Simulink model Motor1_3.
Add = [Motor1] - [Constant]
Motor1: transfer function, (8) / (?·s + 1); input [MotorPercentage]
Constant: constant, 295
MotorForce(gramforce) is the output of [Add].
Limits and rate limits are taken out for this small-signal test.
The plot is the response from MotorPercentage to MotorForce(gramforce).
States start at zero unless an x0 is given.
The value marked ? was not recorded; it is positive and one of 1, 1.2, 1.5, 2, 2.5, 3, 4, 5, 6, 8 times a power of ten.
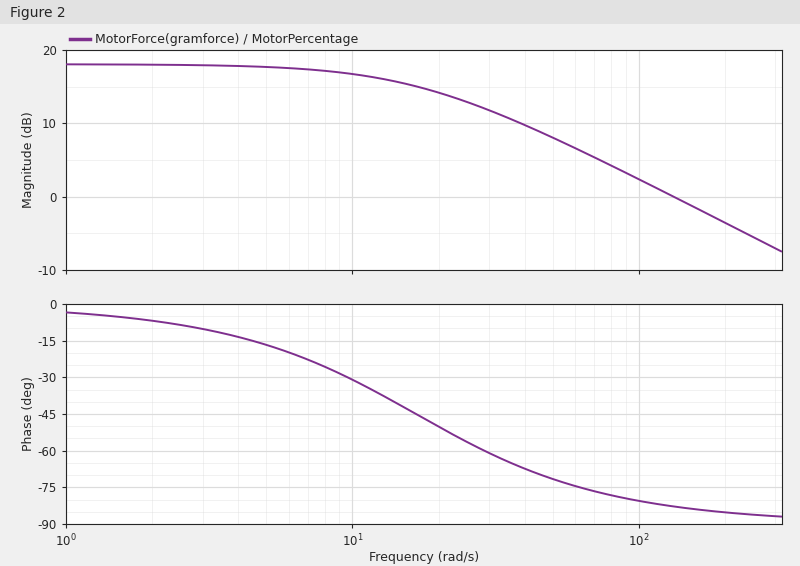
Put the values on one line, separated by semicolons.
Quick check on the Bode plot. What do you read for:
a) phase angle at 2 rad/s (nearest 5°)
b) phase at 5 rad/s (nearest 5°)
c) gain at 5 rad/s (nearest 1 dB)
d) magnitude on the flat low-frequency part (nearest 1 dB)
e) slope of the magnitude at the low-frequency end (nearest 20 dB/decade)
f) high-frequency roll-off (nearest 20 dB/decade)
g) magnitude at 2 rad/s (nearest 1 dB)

-5°; -15°; 18 dB; 18 dB; 0 dB/decade; -20 dB/decade; 18 dB
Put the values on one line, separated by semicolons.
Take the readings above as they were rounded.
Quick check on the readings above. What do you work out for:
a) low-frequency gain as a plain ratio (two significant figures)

7.9
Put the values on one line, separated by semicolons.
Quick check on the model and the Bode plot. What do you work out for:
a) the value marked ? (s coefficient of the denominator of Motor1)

0.06
